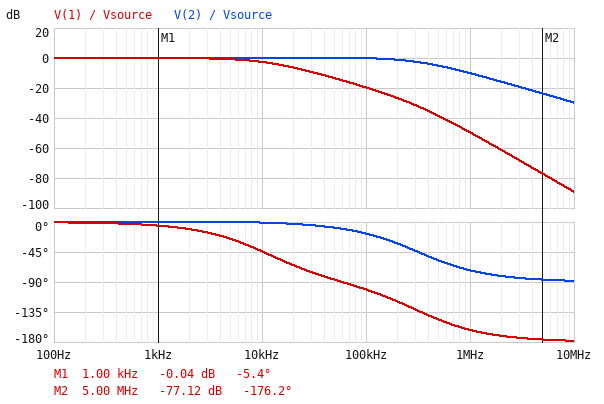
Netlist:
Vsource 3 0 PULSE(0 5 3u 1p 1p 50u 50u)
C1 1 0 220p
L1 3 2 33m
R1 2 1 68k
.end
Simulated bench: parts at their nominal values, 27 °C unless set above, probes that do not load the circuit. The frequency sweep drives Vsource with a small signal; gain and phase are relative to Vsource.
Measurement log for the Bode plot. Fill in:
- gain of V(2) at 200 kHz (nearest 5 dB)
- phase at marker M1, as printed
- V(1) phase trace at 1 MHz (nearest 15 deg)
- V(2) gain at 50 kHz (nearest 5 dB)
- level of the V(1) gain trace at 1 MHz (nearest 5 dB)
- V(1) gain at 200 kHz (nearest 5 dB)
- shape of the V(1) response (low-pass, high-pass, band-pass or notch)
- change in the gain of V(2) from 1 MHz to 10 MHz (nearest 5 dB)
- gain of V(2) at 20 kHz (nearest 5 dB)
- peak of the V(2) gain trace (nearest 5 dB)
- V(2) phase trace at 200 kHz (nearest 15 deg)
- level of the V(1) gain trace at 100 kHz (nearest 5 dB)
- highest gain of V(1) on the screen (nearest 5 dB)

0 dB
-5.4 deg
-165 deg
0 dB
-50 dB
-25 dB
low-pass
-20 dB
0 dB
0 dB
-30 deg
-20 dB
0 dB
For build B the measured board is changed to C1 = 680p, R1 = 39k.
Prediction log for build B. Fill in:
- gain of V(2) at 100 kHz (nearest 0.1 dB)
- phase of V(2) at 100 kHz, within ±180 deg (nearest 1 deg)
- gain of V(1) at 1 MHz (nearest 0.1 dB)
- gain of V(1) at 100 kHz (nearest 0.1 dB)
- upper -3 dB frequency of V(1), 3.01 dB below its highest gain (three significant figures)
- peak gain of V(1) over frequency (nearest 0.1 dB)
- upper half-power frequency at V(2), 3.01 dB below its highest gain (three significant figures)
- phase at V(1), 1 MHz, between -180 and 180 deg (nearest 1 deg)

-0.9 dB
-29 deg
-59.1 dB
-25.3 dB
6.20 kHz
0 dB
185 kHz
-169 deg
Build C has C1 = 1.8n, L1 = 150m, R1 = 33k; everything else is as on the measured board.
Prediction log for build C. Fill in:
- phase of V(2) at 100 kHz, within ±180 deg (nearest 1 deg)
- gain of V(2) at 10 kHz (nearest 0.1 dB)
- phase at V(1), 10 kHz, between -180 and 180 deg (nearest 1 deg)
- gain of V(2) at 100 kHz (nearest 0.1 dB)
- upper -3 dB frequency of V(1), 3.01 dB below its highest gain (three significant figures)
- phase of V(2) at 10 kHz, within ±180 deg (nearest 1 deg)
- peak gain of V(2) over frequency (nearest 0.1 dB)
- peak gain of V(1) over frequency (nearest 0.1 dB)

-72 deg
0.3 dB
-91 deg
-9.5 dB
2.90 kHz
-16 deg
0.5 dB
0 dB
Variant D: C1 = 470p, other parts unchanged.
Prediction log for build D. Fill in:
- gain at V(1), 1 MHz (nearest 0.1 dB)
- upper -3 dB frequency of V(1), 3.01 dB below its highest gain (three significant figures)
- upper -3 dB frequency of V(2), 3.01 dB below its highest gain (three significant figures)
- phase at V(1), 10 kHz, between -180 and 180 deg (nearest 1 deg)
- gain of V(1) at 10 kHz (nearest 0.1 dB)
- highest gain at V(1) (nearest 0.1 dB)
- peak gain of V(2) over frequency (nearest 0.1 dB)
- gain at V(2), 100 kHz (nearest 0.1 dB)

-56.2 dB
5.06 kHz
325 kHz
-65 deg
-6.9 dB
0 dB
0.1 dB
-0.3 dB
